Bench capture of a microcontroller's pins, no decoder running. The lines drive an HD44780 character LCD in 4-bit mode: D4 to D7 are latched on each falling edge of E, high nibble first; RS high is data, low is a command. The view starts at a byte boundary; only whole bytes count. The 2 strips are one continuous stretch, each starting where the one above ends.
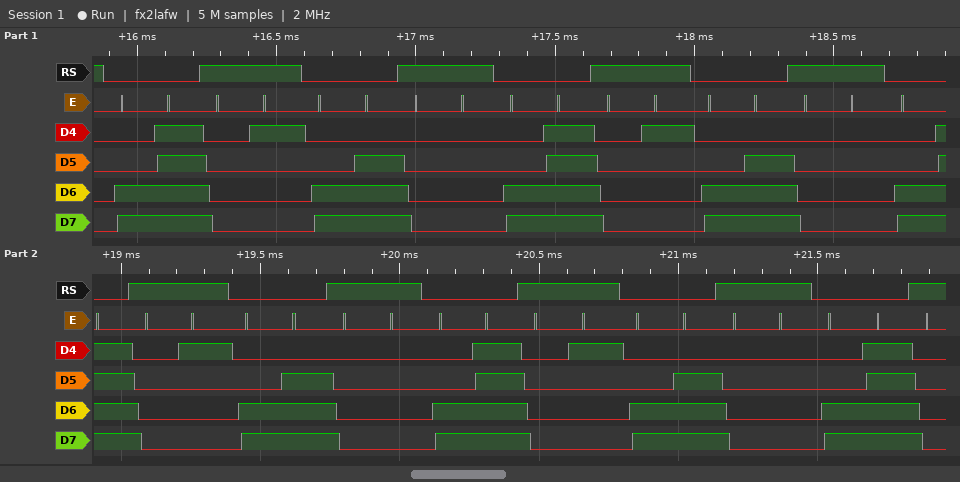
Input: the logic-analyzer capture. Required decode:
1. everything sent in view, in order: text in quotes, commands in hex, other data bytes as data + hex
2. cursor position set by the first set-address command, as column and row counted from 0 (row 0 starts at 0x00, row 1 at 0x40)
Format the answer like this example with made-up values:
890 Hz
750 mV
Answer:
0xCF data 01 0xCE data 00 0xCF data 01 0xCE data 00 0xCF data 01 0xCE data 00 0xCF data 01 0xCE data 00 0xCF
column 15, row 1
